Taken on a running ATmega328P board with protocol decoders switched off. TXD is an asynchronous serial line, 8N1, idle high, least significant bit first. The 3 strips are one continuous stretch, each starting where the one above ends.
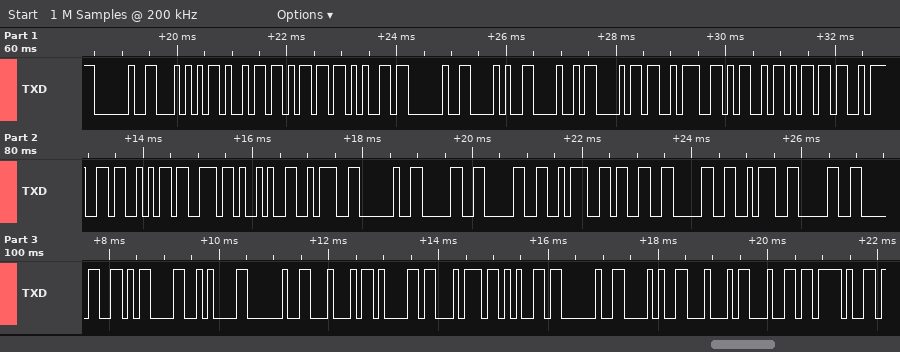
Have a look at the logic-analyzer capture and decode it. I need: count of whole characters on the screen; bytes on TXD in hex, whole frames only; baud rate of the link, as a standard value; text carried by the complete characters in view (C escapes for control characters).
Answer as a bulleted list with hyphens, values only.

- 38
- 20 54 69 6D 65 20 28 48 68 3A 4D 6D 3A 53 73 29 3A 20 30 30 3A 33 30 3A 30 30 0D 0A 20 44 61 74 65 20 28 44 64 2F
- 9600 baud
- " Time (Hh:Mm:Ss): 00:30:00\r\n Date (Dd/"
